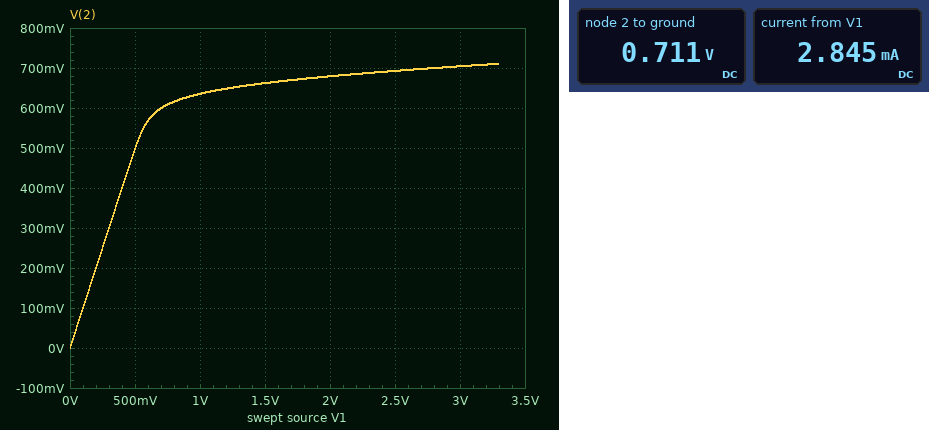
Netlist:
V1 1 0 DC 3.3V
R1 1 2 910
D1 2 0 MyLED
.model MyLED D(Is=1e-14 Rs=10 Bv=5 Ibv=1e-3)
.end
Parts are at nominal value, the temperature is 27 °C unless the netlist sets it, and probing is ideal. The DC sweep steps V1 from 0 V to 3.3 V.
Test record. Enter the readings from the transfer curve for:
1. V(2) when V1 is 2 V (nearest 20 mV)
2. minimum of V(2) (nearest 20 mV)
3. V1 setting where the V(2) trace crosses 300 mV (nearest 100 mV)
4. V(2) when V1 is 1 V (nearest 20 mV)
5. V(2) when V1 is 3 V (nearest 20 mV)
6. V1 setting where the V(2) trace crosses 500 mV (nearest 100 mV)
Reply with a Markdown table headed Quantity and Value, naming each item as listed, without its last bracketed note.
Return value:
| Quantity | Value |
|---|---|
| V(2) when V1 is 2 V | 680 mV |
| minimum of V(2) | 0 V |
| V1 setting where the V(2) trace crosses 300 mV | 300 mV |
| V(2) when V1 is 1 V | 640 mV |
| V(2) when V1 is 3 V | 700 mV |
| V1 setting where the V(2) trace crosses 500 mV | 500 mV |
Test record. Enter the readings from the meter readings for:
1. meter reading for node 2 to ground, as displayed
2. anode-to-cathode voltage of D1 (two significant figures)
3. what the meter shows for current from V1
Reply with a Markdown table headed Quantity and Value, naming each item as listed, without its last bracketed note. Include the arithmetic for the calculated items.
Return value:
| Quantity | Value |
|---|---|
| meter reading for node 2 to ground, as displayed | 0.711 V |
| anode-to-cathode voltage of D1 | 711 mV = 710 mV |
| what the meter shows for current from V1 | 2.845 mA |
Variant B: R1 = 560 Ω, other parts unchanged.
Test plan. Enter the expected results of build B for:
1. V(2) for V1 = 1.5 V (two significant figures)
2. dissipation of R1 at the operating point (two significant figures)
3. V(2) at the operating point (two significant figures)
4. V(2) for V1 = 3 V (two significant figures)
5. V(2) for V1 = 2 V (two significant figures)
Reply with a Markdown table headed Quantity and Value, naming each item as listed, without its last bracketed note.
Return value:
| Quantity | Value |
|---|---|
| V(2) for V1 = 1.5 V | 680 mV |
| dissipation of R1 at the operating point | 12 mW |
| V(2) at the operating point | 740 mV |
| V(2) for V1 = 3 V | 730 mV |
| V(2) for V1 = 2 V | 700 mV |
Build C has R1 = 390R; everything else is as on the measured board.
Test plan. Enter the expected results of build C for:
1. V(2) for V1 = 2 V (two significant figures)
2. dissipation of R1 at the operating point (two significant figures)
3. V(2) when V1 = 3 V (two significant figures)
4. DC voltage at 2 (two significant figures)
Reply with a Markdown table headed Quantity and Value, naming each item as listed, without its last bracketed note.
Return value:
| Quantity | Value |
|---|---|
| V(2) for V1 = 2 V | 720 mV |
| dissipation of R1 at the operating point | 16 mW |
| V(2) when V1 = 3 V | 760 mV |
| DC voltage at 2 | 770 mV |
